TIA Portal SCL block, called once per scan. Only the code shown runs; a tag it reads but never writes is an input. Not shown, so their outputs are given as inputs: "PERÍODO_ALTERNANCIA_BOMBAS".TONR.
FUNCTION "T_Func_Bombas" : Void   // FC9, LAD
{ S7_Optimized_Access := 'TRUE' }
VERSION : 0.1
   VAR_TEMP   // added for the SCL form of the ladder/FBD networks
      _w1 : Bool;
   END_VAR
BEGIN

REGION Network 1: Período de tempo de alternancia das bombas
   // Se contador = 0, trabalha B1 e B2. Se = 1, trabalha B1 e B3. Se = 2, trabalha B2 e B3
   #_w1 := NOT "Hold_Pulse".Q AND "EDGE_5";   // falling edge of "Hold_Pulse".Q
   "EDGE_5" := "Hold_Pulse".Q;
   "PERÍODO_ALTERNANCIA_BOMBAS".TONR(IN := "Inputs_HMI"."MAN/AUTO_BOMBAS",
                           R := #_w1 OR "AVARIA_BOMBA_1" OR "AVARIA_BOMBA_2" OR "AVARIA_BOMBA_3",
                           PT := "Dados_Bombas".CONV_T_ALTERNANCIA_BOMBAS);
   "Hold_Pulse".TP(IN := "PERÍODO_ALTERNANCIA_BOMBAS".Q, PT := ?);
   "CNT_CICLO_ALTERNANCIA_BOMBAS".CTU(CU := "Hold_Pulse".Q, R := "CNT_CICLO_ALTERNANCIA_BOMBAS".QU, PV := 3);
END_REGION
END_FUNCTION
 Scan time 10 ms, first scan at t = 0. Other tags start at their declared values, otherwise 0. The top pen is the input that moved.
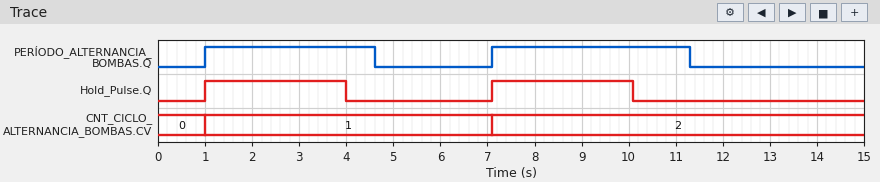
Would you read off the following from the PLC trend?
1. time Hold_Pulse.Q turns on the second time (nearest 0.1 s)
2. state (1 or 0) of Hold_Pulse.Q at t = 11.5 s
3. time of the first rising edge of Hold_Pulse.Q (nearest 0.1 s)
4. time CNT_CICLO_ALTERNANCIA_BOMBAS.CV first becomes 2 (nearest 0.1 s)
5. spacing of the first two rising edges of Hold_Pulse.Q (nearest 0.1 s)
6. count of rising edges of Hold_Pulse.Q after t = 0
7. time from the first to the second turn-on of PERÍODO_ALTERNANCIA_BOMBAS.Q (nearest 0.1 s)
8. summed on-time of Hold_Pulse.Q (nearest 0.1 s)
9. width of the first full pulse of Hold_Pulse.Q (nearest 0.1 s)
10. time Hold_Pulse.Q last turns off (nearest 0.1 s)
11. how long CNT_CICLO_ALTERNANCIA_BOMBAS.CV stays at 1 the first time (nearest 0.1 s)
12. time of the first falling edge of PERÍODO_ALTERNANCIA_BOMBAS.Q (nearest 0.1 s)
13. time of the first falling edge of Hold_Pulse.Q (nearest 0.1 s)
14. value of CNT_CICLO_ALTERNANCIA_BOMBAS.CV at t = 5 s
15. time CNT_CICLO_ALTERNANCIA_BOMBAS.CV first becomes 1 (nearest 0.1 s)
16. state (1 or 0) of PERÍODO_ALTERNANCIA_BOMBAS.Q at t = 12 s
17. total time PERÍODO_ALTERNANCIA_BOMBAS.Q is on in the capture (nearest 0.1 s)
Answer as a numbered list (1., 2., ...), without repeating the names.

1. 7.1 s
2. 0
3. 1.0 s
4. 7.1 s
5. 6.1 s
6. 2
7. 6.1 s
8. 6.0 s
9. 3.0 s
10. 10.1 s
11. 6.1 s
12. 4.6 s
13. 4.0 s
14. 1
15. 1.0 s
16. 0
17. 7.8 s
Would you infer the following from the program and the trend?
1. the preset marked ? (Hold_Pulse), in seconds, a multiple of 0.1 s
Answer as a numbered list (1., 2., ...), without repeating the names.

1. 3.0 s
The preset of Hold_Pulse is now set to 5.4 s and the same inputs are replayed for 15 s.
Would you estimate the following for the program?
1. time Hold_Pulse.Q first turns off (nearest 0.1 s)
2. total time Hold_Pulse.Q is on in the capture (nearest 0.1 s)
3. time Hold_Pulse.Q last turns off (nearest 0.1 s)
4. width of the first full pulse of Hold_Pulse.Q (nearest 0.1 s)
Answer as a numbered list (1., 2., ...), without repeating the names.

1. 6.4 s
2. 10.8 s
3. 12.5 s
4. 5.4 s
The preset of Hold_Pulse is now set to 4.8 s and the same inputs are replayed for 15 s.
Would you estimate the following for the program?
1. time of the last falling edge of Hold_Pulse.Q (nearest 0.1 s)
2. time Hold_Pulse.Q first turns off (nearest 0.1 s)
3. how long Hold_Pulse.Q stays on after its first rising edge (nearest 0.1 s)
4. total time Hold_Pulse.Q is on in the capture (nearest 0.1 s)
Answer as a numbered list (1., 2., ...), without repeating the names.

1. 11.9 s
2. 5.8 s
3. 4.8 s
4. 9.6 s
